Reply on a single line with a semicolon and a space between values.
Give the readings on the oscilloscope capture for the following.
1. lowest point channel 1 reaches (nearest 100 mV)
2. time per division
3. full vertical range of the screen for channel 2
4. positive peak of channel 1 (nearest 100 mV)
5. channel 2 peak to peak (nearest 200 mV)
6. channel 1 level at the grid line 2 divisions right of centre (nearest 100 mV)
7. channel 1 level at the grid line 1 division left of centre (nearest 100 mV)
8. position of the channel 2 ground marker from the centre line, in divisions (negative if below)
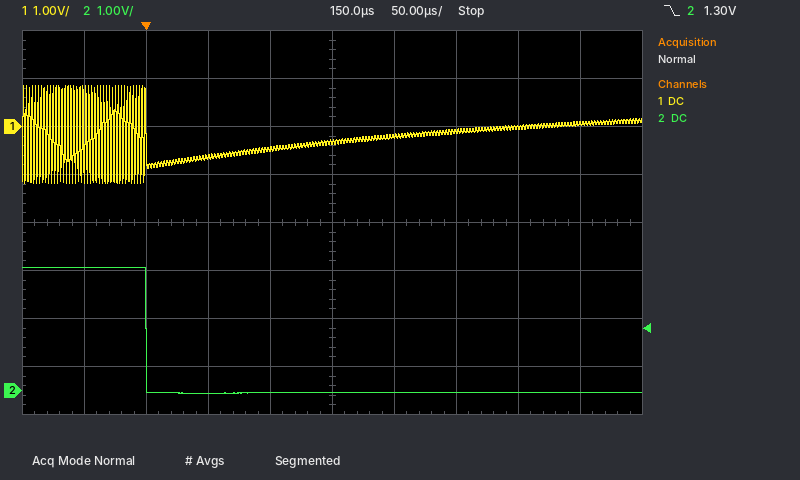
-1.2 V; 50 µs; 8 V; 900 mV; 2.6 V; -100 mV; -500 mV; -3.5 div
